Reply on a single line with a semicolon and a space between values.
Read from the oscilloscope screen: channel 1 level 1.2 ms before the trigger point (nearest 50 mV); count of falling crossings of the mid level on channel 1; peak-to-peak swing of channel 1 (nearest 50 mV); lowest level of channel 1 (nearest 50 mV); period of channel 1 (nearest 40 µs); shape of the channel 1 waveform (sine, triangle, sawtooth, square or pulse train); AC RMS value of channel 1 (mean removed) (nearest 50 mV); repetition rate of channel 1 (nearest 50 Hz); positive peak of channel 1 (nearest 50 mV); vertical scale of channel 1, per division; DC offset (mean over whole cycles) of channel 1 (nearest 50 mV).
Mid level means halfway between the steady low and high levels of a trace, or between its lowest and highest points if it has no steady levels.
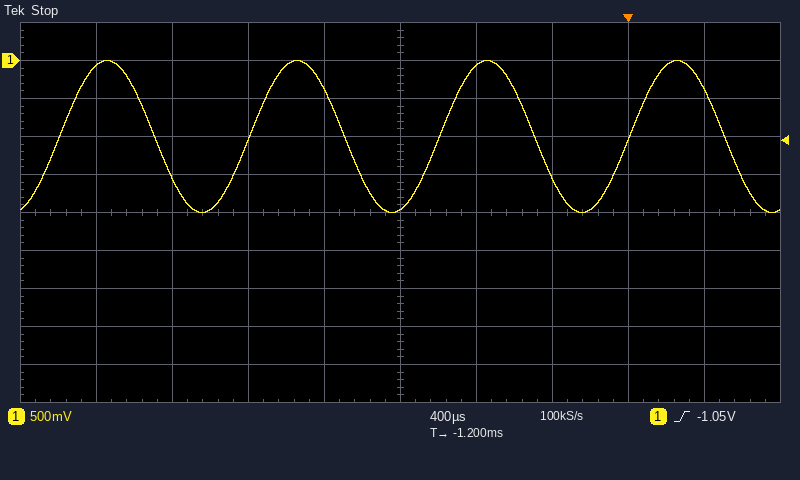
-1.95 V; 4; 2.00 V; -2.00 V; 1.00 ms; sine; 700 mV; 1.00 kHz; 0 mV; 500 mV; -1.00 V
